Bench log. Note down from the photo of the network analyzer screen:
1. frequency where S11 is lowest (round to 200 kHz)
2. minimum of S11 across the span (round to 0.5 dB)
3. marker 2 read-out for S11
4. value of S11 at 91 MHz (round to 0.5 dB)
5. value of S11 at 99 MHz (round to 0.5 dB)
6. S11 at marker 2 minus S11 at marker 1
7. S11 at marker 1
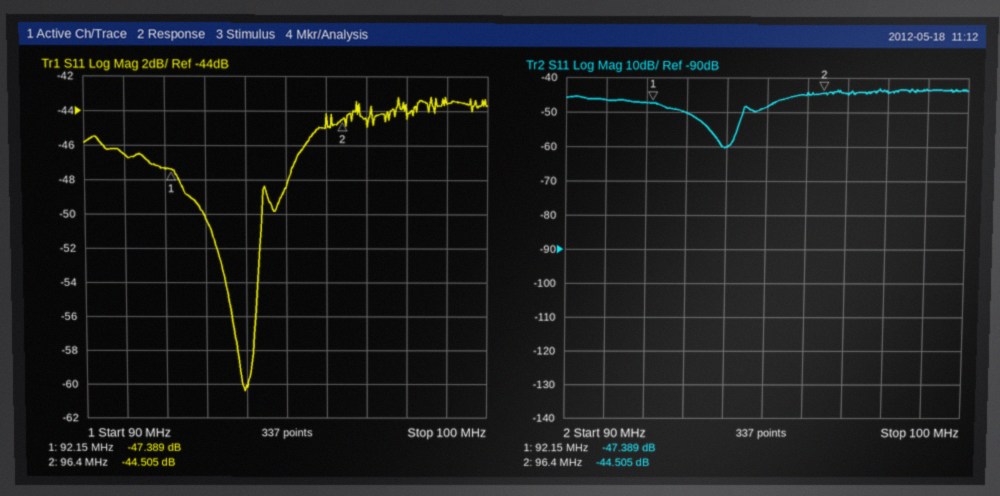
94.0 MHz
-60.5 dB
-44.505 dB
-46.5 dB
-43.5 dB
2.884 dB
-47.389 dB
